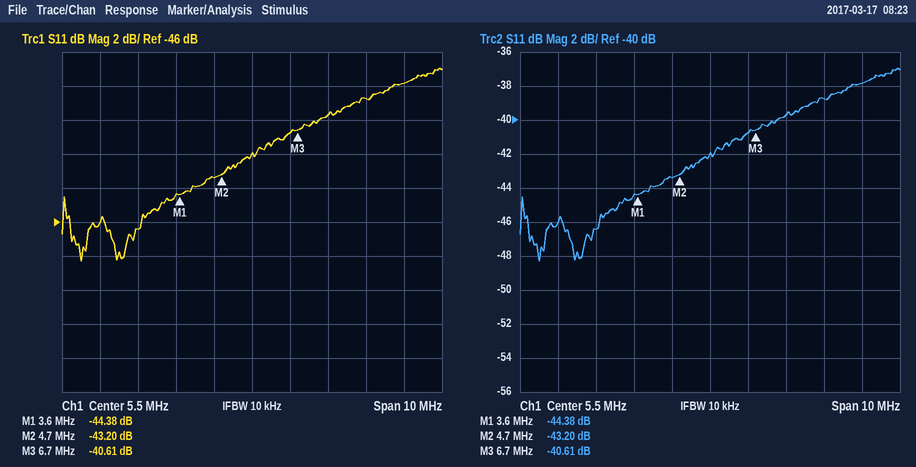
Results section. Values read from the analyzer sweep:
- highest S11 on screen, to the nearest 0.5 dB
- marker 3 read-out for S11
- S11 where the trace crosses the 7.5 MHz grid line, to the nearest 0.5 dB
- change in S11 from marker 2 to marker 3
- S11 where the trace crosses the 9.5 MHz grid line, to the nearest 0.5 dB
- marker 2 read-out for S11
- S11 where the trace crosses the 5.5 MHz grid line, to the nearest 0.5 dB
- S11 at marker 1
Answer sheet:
-37.0 dB
-40.61 dB
-39.5 dB
2.59 dB
-38.0 dB
-43.20 dB
-42.0 dB
-44.38 dB
